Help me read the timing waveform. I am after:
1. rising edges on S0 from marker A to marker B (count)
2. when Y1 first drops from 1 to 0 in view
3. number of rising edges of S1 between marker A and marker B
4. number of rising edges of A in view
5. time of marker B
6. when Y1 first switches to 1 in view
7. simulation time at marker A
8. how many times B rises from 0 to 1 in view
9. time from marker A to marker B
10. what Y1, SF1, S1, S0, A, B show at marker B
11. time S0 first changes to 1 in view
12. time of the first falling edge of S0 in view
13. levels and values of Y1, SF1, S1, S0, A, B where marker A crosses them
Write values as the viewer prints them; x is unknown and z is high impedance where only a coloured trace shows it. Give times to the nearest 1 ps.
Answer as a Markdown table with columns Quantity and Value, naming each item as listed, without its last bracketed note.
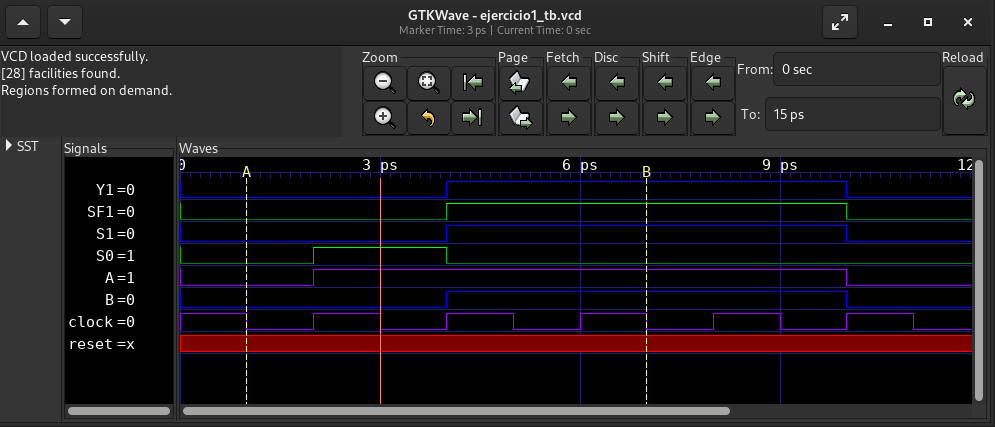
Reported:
| Quantity | Value |
|---|---|
| rising edges on S0 from marker A to marker B | 1 |
| when Y1 first drops from 1 to 0 in view | 10 ps |
| number of rising edges of S1 between marker A and marker B | 1 |
| number of rising edges of A in view | 1 |
| time of marker B | 7 ps |
| when Y1 first switches to 1 in view | 4 ps |
| simulation time at marker A | 1 ps |
| how many times B rises from 0 to 1 in view | 1 |
| time from marker A to marker B | 6 ps |
| what Y1, SF1, S1, S0, A, B show at marker B | Y1=1, SF1=1, S1=1, S0=0, A=1, B=1 |
| time S0 first changes to 1 in view | 2 ps |
| time of the first falling edge of S0 in view | 4 ps |
| levels and values of Y1, SF1, S1, S0, A, B where marker A crosses them | Y1=0, SF1=0, S1=0, S0=0, A=0, B=0 |
